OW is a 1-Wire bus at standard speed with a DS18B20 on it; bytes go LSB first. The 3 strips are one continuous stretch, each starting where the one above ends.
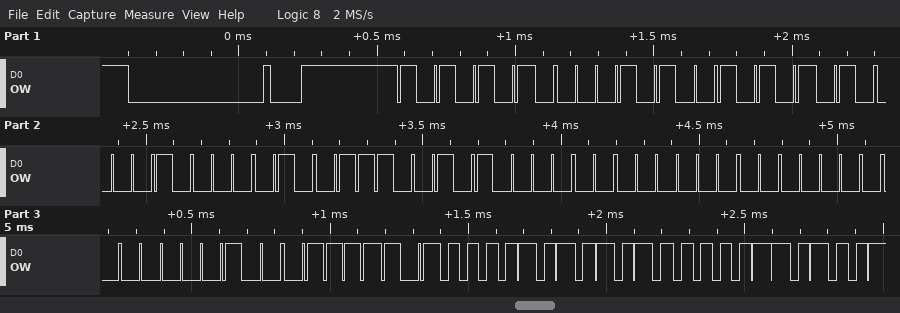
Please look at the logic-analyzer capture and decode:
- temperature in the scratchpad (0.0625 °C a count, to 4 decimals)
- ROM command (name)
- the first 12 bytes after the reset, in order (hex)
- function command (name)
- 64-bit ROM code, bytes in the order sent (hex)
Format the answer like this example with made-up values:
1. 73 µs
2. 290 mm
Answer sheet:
1. 85.0000 °C
2. Match ROM
3. 55 28 55 08 72 0A 00 00 20 BE 50 05
4. Read Scratchpad
5. 28 55 08 72 0A 00 00 20
